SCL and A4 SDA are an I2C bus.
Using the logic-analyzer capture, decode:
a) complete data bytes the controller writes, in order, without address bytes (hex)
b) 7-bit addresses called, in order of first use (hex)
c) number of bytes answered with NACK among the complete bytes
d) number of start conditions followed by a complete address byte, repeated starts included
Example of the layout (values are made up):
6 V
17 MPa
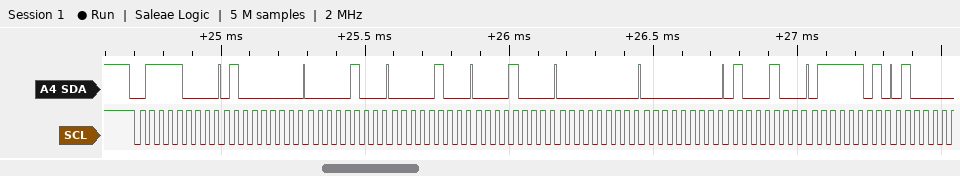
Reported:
40 04 04 08 00 00 44 7D
0x3C
0
1
